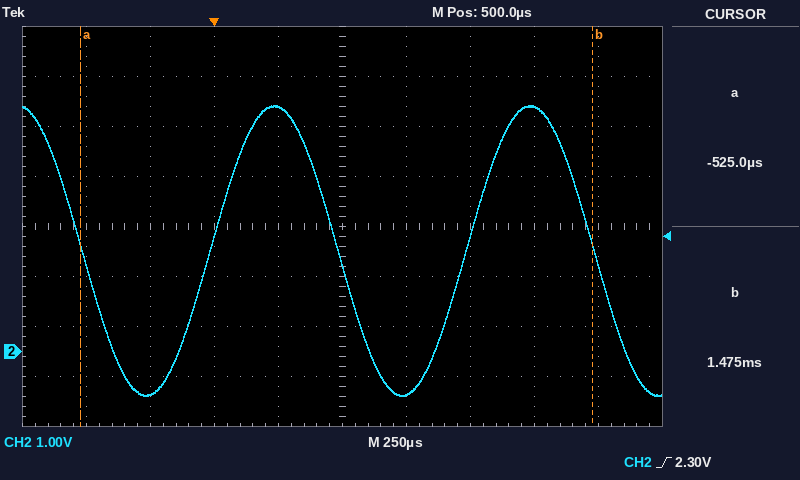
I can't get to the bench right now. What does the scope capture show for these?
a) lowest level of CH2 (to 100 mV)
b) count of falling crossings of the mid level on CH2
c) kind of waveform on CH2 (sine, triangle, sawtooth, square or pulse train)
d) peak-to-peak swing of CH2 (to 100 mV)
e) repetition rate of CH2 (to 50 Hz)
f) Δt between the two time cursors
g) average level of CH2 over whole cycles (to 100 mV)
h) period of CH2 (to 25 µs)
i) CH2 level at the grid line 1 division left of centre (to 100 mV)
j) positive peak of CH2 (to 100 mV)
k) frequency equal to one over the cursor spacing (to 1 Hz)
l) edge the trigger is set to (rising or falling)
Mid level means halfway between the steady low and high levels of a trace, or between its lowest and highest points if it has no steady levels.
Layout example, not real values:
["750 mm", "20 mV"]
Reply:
["-900 mV", "3", "sine", "5.8 V", "1.00 kHz", "2.000 ms", "2.0 V", "1.000 ms", "4.9 V", "4.9 V", "500 Hz", "rising"]
